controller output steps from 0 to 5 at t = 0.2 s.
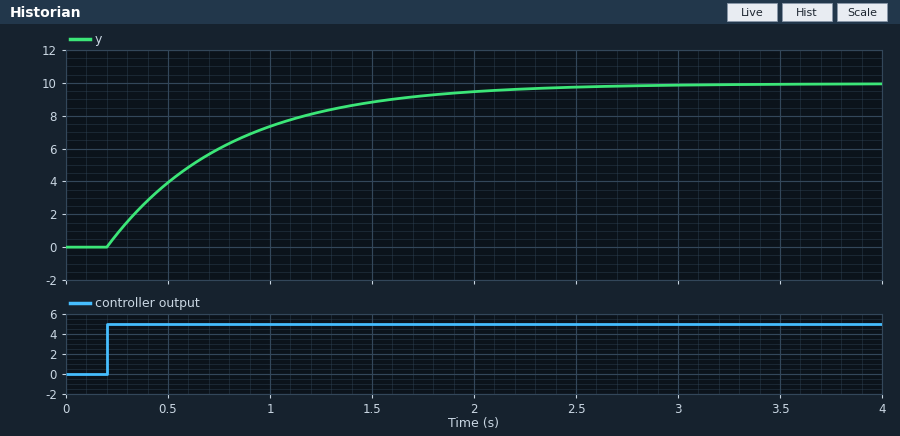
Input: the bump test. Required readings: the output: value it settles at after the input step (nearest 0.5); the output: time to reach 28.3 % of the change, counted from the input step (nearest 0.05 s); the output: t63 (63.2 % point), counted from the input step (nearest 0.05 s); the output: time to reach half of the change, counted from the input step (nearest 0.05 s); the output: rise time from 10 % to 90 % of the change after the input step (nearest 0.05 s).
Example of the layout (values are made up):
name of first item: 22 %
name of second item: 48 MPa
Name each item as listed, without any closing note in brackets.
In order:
the output: value it settles at after the input step: 10.0
the output: time to reach 28.3 % of the change, counted from the input step: 0.20 s
the output: t63 (63.2 % point), counted from the input step: 0.60 s
the output: time to reach half of the change, counted from the input step: 0.40 s
the output: rise time from 10 % to 90 % of the change after the input step: 1.30 s
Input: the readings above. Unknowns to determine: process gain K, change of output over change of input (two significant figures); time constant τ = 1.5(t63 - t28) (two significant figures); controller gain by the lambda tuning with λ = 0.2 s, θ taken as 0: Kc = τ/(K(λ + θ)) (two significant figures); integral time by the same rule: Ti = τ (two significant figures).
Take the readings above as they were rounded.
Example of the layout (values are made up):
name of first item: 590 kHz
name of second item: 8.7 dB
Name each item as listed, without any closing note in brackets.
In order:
process gain K, change of output over change of input: 2.0
time constant τ = 1.5(t63 - t28): 0.60 s
controller gain by the lambda tuning with λ = 0.2 s, θ taken as 0: Kc = τ/(K(λ + θ)): 1.5
integral time by the same rule: Ti = τ: 0.60 s
